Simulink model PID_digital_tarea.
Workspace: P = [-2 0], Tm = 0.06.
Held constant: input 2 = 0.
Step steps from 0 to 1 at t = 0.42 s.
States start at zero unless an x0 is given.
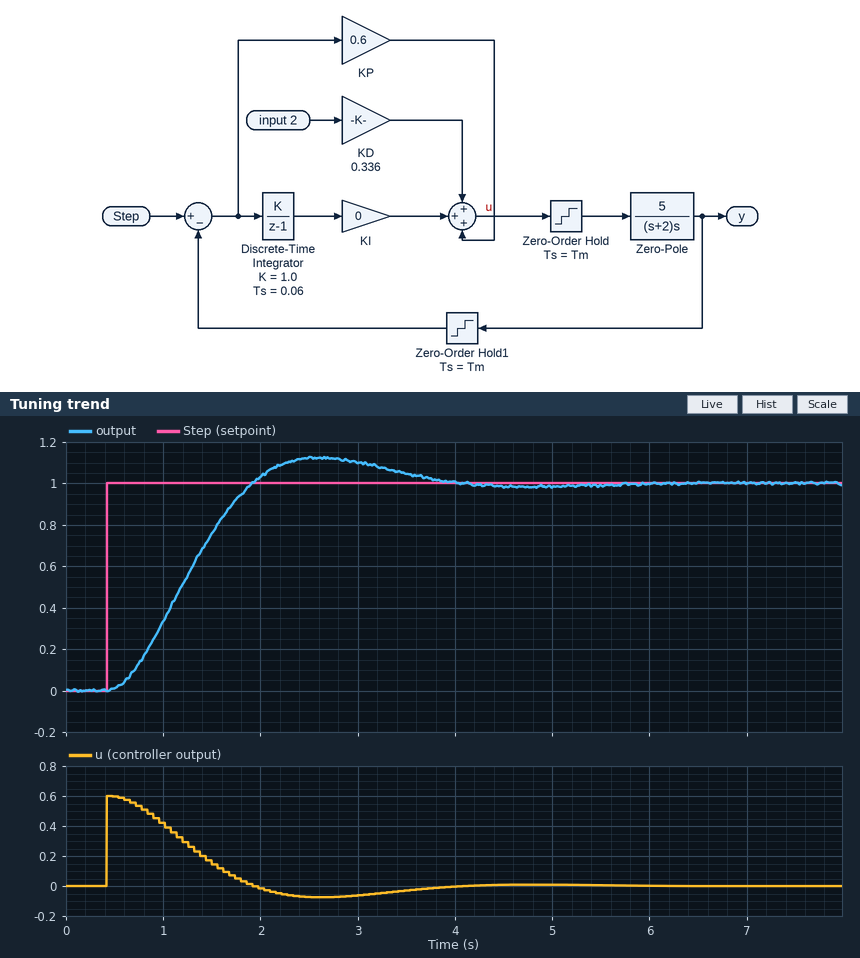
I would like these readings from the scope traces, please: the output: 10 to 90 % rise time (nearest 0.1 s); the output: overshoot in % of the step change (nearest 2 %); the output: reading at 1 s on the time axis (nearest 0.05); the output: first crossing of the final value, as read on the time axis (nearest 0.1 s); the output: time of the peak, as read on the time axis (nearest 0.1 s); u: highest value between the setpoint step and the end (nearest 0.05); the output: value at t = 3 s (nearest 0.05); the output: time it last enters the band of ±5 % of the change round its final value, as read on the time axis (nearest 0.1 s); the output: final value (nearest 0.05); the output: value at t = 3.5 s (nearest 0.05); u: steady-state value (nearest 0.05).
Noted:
1.0 s
12 %
0.35
1.9 s
2.6 s
0.60
1.10
3.5 s
1.00
1.05
0.00
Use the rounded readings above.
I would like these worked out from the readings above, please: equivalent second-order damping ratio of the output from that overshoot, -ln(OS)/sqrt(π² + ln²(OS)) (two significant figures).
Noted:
0.56
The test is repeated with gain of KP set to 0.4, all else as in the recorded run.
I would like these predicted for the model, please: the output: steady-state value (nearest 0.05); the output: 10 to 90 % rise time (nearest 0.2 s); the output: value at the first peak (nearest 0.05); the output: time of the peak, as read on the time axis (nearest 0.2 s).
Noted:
1.00
1.4 s
1.05
3.4 s
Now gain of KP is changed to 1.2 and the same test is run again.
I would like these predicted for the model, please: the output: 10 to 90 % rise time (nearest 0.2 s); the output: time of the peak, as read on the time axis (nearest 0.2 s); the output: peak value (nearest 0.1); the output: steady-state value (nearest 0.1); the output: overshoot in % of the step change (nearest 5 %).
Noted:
0.6 s
1.8 s
1.3
1.0
30 %
